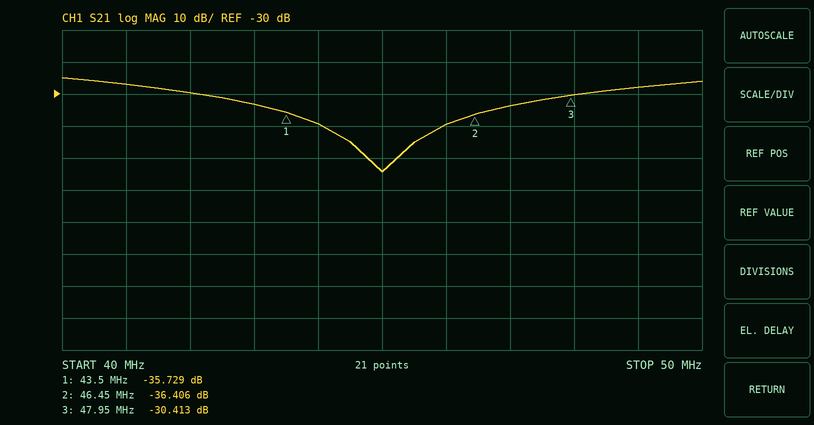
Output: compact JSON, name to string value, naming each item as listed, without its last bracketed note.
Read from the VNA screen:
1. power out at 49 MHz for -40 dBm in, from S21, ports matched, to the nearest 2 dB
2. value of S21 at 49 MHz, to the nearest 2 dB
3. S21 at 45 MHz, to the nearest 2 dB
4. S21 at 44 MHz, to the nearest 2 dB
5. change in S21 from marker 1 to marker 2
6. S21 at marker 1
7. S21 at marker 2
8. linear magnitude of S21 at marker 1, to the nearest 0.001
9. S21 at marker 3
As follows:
{"power out at 49 MHz for -40 dBm in, from S21, ports matched, to the nearest 2 dB": "-68 dBm", "value of S21 at 49 MHz, to the nearest 2 dB": "-28 dB", "S21 at 45 MHz, to the nearest 2 dB": "-54 dB", "S21 at 44 MHz, to the nearest 2 dB": "-40 dB", "change in S21 from marker 1 to marker 2": "-0.677 dB", "S21 at marker 1": "-35.729 dB", "S21 at marker 2": "-36.406 dB", "linear magnitude of S21 at marker 1, to the nearest 0.001": "0.016", "S21 at marker 3": "-30.413 dB"}
